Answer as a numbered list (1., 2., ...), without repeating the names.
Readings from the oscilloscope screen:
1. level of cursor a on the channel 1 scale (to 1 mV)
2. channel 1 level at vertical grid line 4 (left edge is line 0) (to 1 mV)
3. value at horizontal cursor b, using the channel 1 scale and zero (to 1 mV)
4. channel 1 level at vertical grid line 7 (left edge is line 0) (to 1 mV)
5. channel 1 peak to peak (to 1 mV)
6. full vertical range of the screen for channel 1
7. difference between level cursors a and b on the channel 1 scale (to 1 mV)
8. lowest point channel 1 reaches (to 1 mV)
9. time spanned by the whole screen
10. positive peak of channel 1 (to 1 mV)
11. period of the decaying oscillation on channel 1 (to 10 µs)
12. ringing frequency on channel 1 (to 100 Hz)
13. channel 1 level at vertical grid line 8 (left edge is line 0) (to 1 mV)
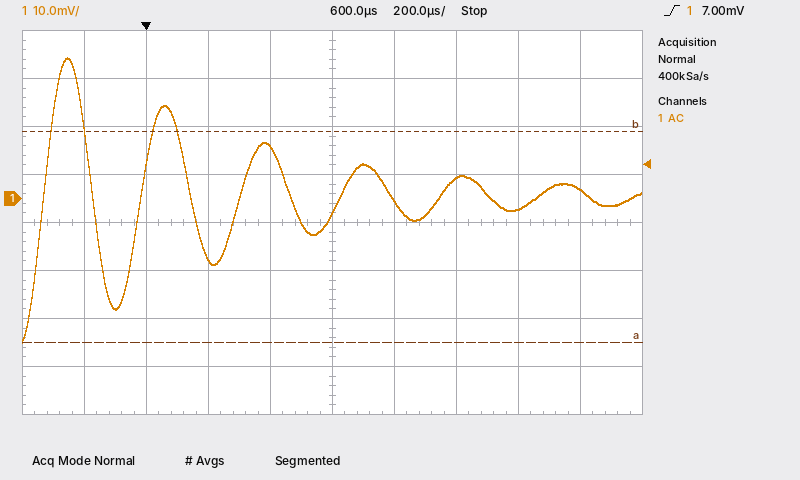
1. -30 mV
2. 11 mV
3. 14 mV
4. 4 mV
5. 59 mV
6. 80 mV
7. 44 mV
8. -30 mV
9. 2 ms
10. 29 mV
11. 320 µs
12. 3.1 kHz
13. -2 mV
